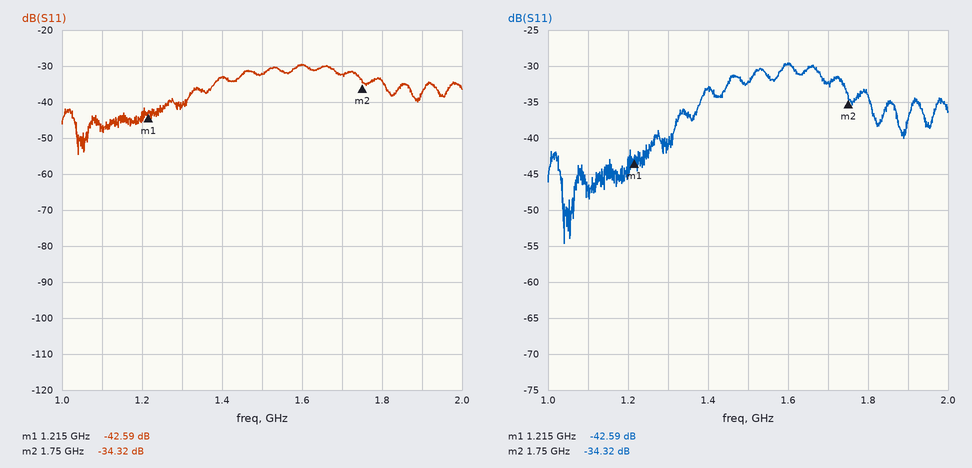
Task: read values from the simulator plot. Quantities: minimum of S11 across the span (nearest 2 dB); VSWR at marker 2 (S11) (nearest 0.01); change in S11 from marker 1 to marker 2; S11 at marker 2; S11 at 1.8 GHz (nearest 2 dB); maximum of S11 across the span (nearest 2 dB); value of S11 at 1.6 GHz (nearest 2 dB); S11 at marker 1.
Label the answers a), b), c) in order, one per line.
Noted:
a) -54 dB
b) 1.04
c) 8.27 dB
d) -34.32 dB
e) -34 dB
f) -30 dB
g) -30 dB
h) -42.59 dB
